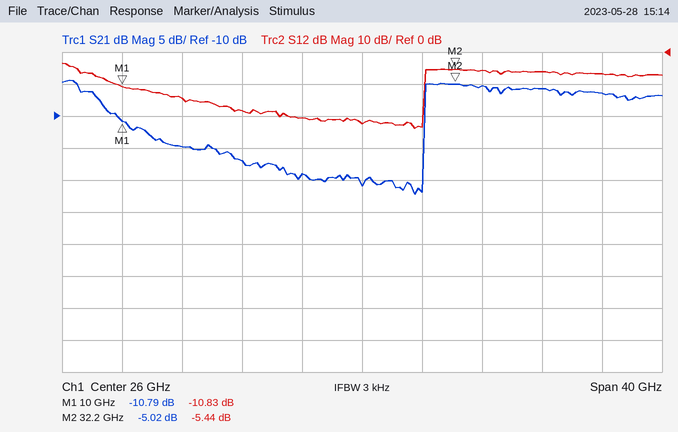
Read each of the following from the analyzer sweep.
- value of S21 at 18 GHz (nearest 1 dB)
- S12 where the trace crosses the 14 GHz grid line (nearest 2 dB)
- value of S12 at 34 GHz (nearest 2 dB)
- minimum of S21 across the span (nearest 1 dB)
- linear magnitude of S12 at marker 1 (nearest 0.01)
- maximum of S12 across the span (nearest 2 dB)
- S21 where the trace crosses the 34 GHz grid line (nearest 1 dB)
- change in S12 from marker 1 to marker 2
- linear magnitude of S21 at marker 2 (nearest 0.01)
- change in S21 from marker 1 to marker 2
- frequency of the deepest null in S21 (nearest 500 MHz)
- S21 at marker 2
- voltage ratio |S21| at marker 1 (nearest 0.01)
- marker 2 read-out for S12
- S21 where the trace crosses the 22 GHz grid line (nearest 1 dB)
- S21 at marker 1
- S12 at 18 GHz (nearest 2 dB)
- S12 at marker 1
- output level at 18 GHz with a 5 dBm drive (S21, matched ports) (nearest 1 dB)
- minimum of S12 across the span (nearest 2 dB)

-17 dB
-14 dB
-6 dB
-22 dB
0.29
-4 dB
-5 dB
5.39 dB
0.56
5.77 dB
29.5 GHz
-5.02 dB
0.29
-5.44 dB
-19 dB
-10.79 dB
-18 dB
-10.83 dB
-12 dBm
-24 dB
